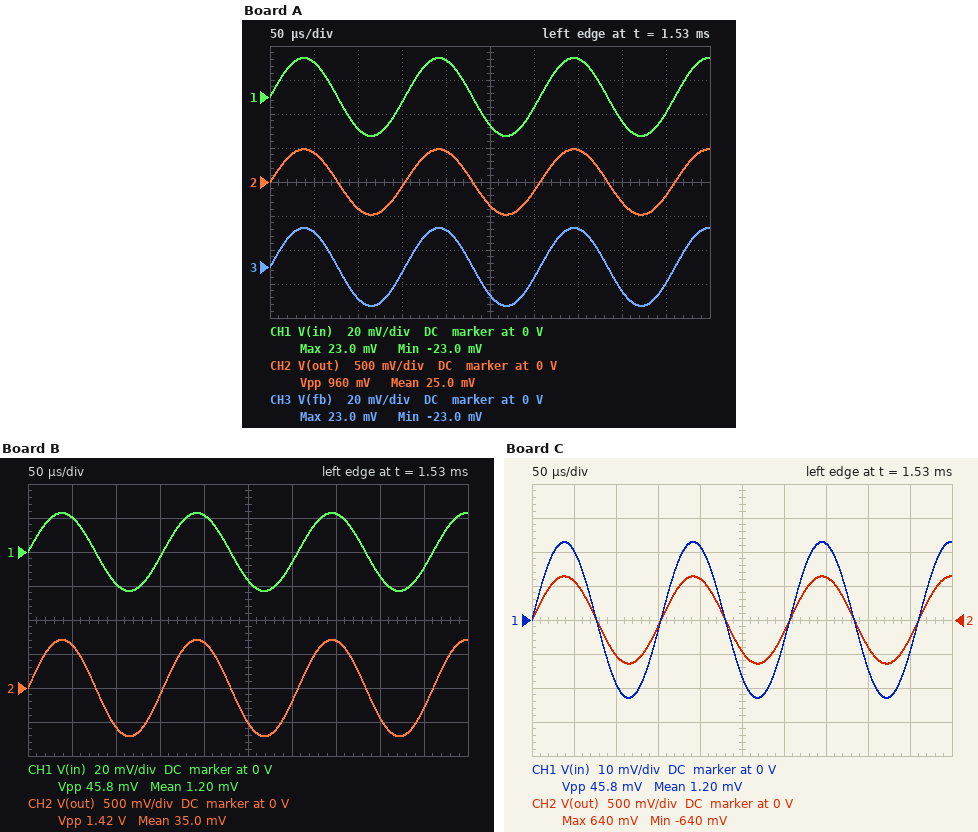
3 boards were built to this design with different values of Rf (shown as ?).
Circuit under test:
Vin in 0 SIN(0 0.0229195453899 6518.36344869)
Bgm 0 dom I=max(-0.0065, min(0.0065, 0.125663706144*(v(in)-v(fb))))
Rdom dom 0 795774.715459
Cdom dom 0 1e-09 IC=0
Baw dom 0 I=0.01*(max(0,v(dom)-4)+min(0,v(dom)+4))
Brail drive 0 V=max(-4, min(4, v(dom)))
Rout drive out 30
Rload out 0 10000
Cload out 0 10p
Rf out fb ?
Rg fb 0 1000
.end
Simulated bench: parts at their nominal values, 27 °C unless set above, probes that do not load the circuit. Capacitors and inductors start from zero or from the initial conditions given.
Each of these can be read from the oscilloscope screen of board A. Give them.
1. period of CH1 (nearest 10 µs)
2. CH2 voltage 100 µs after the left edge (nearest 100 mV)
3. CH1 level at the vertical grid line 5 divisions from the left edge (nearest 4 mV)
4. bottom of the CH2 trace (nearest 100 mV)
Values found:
150 µs
-400 mV
-16 mV
-500 mV
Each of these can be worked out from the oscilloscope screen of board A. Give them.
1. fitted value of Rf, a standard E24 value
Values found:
20 kΩ
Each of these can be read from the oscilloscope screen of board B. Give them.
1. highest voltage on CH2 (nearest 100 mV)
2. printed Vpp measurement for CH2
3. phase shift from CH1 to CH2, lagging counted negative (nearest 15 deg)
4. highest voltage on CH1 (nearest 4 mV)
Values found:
700 mV
1.42 V
0 deg
24 mV
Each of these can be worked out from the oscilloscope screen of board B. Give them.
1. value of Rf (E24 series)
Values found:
30 kΩ
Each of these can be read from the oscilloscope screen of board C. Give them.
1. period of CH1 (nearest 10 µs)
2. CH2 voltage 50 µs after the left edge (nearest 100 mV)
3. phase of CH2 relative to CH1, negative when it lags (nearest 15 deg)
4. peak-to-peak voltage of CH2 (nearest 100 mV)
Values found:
150 µs
600 mV
0 deg
1.3 V
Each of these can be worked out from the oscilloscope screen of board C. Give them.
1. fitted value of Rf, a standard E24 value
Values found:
27 kΩ
